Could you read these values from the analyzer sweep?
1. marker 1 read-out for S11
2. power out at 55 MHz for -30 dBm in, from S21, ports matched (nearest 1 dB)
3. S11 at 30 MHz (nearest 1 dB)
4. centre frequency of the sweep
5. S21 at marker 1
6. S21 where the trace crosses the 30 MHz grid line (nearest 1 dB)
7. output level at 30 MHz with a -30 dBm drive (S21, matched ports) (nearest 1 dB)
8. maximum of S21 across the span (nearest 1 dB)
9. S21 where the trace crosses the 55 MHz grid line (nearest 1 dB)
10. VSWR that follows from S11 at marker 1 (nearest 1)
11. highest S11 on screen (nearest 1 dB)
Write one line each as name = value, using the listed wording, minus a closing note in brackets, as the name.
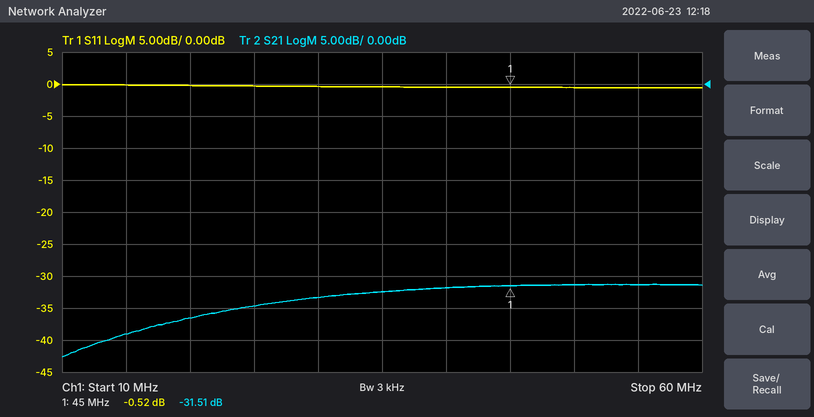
marker 1 read-out for S11 = -0.52 dB
power out at 55 MHz for -30 dBm in, from S21, ports matched = -61 dBm
S11 at 30 MHz = 0 dB
centre frequency of the sweep = 35 MHz
S21 at marker 1 = -31.51 dB
S21 where the trace crosses the 30 MHz grid line = -33 dB
output level at 30 MHz with a -30 dBm drive (S21, matched ports) = -63 dBm
maximum of S21 across the span = -31 dB
S21 where the trace crosses the 55 MHz grid line = -31 dB
VSWR that follows from S11 at marker 1 = 33
highest S11 on screen = 0 dB
